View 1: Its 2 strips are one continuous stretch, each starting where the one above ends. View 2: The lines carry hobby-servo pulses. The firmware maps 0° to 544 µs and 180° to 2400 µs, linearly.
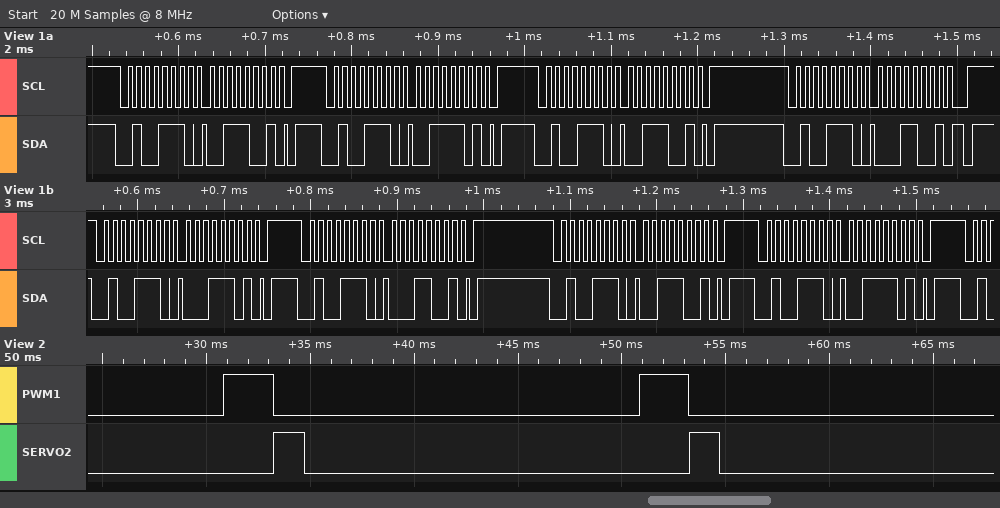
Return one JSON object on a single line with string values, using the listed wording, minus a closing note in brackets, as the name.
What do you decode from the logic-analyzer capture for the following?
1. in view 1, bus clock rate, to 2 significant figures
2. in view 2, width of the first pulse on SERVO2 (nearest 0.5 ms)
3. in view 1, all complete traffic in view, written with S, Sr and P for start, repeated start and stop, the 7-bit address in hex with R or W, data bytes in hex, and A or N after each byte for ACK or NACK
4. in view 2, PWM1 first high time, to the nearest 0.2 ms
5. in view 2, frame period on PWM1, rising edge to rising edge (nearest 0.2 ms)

{"in view 1, bus clock rate, to 2 significant figures": "100 kHz", "in view 2, width of the first pulse on SERVO2": "1.5 ms", "in view 1, all complete traffic in view, written with S, Sr and P for start, repeated start and stop, the 7-bit address in hex with R or W, data bytes in hex, and A or N after each byte for ACK or NACK": "S 27W A 39 A P S 27W A 3D A P S 27W A 39 A P S 27W A 19 A P S 27W A 1D A P S 27W A 19 A P S 27W A 39 A P S 27W A 3D A P", "in view 2, PWM1 first high time, to the nearest 0.2 ms": "2.4 ms", "in view 2, frame period on PWM1, rising edge to rising edge": "20.0 ms"}
